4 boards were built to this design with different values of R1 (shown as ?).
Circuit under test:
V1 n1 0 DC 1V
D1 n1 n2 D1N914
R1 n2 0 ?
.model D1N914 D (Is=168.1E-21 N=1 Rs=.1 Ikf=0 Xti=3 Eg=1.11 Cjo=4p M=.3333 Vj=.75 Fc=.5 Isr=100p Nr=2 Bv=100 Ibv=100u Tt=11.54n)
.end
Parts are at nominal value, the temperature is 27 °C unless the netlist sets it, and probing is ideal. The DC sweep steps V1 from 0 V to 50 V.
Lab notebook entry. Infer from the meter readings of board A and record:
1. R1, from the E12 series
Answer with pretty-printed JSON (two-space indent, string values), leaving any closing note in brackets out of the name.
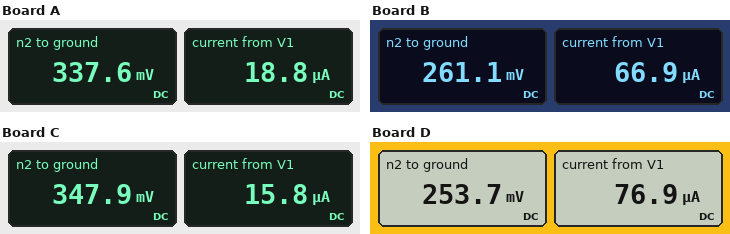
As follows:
{
  "R1, from the E12 series": "18 kΩ"
}
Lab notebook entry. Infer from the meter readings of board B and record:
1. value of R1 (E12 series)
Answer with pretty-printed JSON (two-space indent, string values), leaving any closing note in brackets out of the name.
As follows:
{
  "value of R1": "3.9 kΩ"
}
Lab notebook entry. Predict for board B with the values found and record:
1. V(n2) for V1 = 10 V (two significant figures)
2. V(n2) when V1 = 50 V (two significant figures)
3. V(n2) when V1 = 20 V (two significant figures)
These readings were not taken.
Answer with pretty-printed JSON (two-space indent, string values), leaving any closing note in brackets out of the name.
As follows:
{
  "V(n2) for V1 = 10 V": "9.1 V",
  "V(n2) when V1 = 50 V": "49 V",
  "V(n2) when V1 = 20 V": "19 V"
}
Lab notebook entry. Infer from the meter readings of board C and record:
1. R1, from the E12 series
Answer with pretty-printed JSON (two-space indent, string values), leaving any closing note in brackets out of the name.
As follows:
{
  "R1, from the E12 series": "22 kΩ"
}
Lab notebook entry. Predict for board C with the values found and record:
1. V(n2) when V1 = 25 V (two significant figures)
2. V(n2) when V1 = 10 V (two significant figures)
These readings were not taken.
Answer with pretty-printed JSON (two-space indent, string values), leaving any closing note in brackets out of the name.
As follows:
{
  "V(n2) when V1 = 25 V": "24 V",
  "V(n2) when V1 = 10 V": "9.2 V"
}
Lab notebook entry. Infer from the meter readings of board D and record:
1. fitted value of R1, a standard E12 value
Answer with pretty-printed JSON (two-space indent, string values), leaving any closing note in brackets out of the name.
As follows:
{
  "fitted value of R1, a standard E12 value": "3.3 kΩ"
}
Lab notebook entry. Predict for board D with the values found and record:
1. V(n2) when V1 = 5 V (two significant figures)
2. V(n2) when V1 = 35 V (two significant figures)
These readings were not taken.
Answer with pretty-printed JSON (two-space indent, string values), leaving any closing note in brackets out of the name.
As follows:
{
  "V(n2) when V1 = 5 V": "4.1 V",
  "V(n2) when V1 = 35 V": "34 V"
}
